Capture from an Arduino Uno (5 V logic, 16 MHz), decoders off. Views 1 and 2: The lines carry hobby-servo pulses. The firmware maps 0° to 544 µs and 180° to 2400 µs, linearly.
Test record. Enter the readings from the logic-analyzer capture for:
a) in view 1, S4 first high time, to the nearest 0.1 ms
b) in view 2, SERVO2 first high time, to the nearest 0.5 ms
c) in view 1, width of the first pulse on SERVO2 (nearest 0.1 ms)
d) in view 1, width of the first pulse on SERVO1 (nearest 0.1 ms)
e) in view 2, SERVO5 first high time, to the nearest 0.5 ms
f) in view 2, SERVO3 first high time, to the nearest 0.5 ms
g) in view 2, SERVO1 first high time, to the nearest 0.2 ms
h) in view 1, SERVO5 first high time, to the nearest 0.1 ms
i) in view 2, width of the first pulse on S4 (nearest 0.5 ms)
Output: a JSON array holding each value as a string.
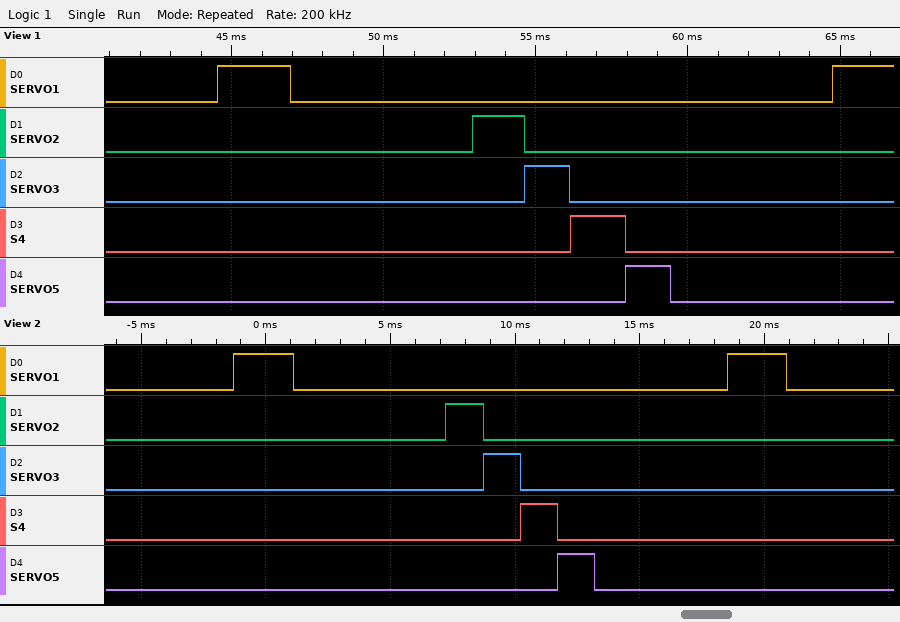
["1.8 ms", "1.5 ms", "1.7 ms", "2.4 ms", "1.5 ms", "1.5 ms", "2.4 ms", "1.5 ms", "1.5 ms"]
